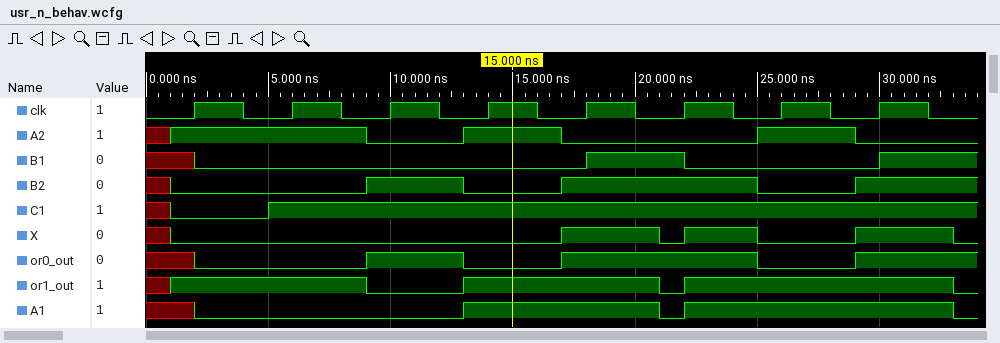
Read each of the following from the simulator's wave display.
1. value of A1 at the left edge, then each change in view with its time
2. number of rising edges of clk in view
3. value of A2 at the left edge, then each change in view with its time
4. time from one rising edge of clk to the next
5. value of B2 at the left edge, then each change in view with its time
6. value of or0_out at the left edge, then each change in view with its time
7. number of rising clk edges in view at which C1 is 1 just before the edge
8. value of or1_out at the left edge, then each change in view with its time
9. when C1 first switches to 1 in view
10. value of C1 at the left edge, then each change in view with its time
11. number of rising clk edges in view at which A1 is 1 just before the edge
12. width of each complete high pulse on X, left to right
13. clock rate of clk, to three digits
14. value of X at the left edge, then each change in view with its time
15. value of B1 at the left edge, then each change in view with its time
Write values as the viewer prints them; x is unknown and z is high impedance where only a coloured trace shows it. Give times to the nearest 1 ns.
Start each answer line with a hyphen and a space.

- x, 0 at 2 ns, 1 at 13 ns, 0 at 21 ns, 1 at 22 ns, 0 at 33 ns
- 8
- x, 1 at 1 ns, 0 at 9 ns, 1 at 13 ns, 0 at 17 ns, 1 at 25 ns, 0 at 29 ns
- 4 ns
- x, 0 at 1 ns, 1 at 9 ns, 0 at 13 ns, 1 at 17 ns, 0 at 25 ns, 1 at 29 ns
- x, 0 at 2 ns, 1 at 9 ns, 0 at 13 ns, 1 at 17 ns, 0 at 25 ns, 1 at 29 ns
- 7
- x, 1 at 1 ns, 0 at 9 ns, 1 at 13 ns, 0 at 21 ns, 1 at 22 ns, 0 at 33 ns
- 5 ns
- x, 0 at 1 ns, 1 at 5 ns
- 4
- 4 ns, 3 ns, 4 ns
- 250 MHz
- x, 0 at 1 ns, 1 at 17 ns, 0 at 21 ns, 1 at 22 ns, 0 at 25 ns, 1 at 29 ns, 0 at 33 ns
- x, 0 at 2 ns, 1 at 18 ns, 0 at 22 ns, 1 at 30 ns
